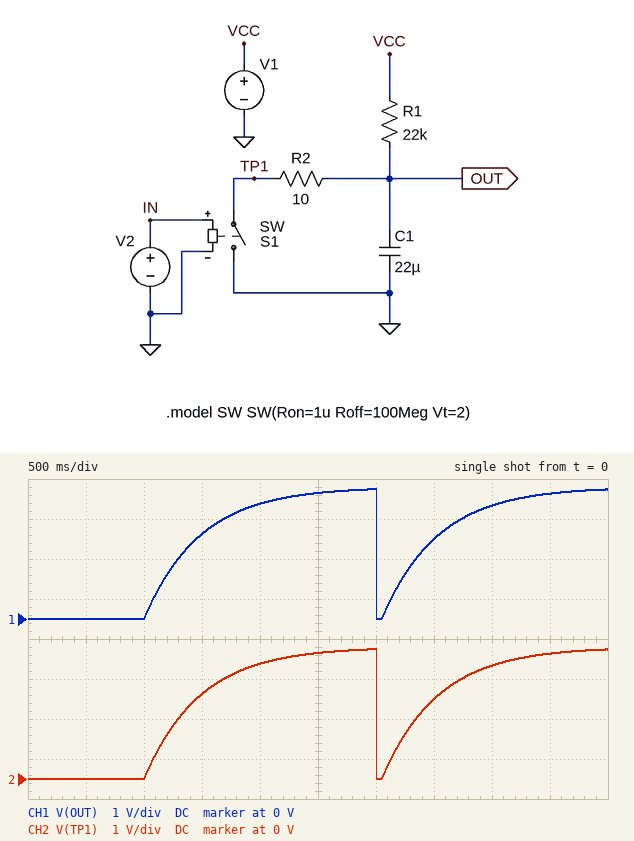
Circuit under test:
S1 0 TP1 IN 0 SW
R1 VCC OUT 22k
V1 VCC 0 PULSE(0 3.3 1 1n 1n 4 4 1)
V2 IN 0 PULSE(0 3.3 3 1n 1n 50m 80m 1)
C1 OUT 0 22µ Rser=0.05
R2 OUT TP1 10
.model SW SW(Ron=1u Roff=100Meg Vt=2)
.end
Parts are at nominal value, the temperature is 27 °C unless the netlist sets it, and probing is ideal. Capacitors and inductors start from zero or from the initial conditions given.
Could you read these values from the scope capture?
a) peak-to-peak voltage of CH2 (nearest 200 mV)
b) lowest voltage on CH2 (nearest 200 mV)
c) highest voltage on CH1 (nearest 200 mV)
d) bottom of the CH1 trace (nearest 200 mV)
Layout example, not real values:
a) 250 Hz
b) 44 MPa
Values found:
a) 3.2 V
b) 0 V
c) 3.2 V
d) 0 V
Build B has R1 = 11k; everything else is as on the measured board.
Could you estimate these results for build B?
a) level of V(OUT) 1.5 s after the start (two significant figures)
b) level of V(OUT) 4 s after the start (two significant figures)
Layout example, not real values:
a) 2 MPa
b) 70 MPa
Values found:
a) 2.9 V
b) 3.2 V
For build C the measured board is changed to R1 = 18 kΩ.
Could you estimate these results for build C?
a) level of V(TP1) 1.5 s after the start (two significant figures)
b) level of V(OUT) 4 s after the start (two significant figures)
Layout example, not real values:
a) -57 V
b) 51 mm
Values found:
a) 2.4 V
b) 3.0 V
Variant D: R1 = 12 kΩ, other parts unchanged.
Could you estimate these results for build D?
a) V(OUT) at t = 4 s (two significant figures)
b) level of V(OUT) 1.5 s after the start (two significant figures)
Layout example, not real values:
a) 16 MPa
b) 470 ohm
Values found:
a) 3.2 V
b) 2.8 V
